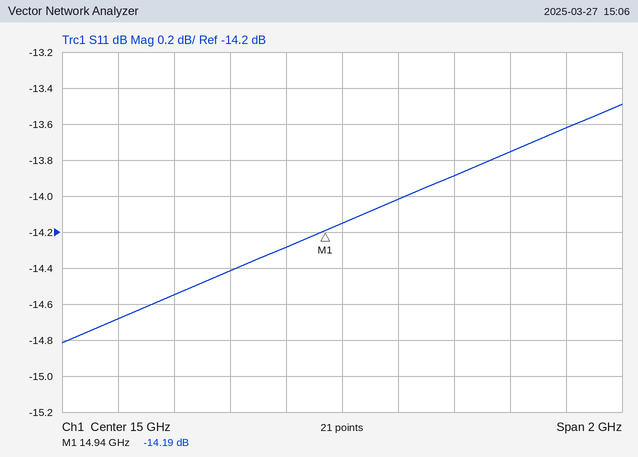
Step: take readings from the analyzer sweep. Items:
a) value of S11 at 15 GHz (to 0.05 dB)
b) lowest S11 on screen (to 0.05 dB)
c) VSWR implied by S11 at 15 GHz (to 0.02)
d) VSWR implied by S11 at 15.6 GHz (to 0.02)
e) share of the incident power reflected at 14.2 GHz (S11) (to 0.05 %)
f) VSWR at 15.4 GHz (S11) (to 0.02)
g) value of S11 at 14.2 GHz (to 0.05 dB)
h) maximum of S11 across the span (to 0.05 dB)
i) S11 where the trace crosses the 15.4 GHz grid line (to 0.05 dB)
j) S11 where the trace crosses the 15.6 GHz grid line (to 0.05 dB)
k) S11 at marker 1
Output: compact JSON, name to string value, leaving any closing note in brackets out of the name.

{"value of S11 at 15 GHz": "-14.15 dB", "lowest S11 on screen": "-14.80 dB", "VSWR implied by S11 at 15 GHz": "1.48", "VSWR implied by S11 at 15.6 GHz": "1.52", "share of the incident power reflected at 14.2 GHz (S11)": "3.40 %", "VSWR at 15.4 GHz (S11)": "1.50", "value of S11 at 14.2 GHz": "-14.70 dB", "maximum of S11 across the span": "-13.50 dB", "S11 where the trace crosses the 15.4 GHz grid line": "-13.90 dB", "S11 where the trace crosses the 15.6 GHz grid line": "-13.75 dB", "S11 at marker 1": "-14.19 dB"}
